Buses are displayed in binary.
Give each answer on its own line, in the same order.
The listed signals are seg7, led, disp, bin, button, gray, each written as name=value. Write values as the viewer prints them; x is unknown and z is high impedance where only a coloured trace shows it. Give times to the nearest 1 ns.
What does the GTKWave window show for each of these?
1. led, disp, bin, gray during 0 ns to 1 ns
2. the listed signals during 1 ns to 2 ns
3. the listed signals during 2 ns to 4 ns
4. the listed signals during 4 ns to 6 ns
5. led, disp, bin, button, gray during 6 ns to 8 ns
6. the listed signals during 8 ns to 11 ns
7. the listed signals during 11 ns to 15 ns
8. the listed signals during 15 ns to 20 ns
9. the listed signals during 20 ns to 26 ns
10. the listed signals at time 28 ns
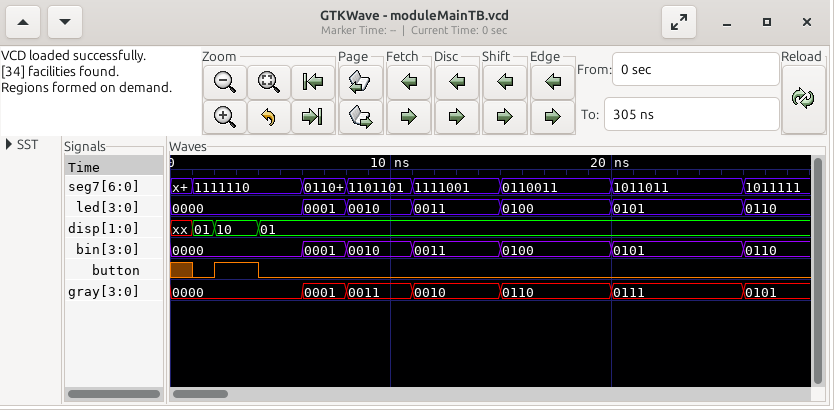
led=0000, disp=xx, bin=0000, gray=0000
seg7=1111110, led=0000, disp=01, bin=0000, button=0, gray=0000
seg7=1111110, led=0000, disp=10, bin=0000, button=1, gray=0000
seg7=1111110, led=0000, disp=01, bin=0000, button=0, gray=0000
led=0001, disp=01, bin=0001, button=0, gray=0001
seg7=1101101, led=0010, disp=01, bin=0010, button=0, gray=0011
seg7=1111001, led=0011, disp=01, bin=0011, button=0, gray=0010
seg7=0110011, led=0100, disp=01, bin=0100, button=0, gray=0110
seg7=1011011, led=0101, disp=01, bin=0101, button=0, gray=0111
seg7=1011111, led=0110, disp=01, bin=0110, button=0, gray=0101
